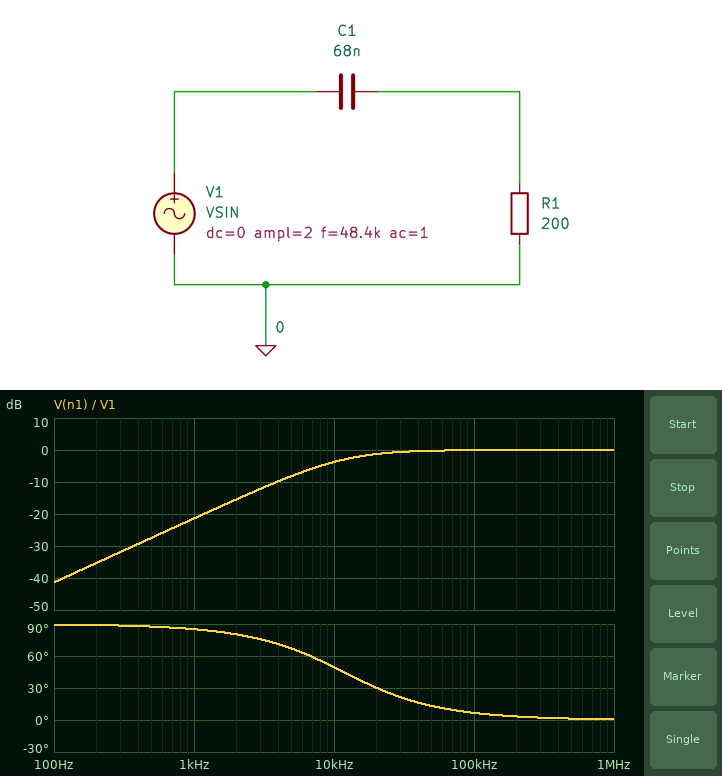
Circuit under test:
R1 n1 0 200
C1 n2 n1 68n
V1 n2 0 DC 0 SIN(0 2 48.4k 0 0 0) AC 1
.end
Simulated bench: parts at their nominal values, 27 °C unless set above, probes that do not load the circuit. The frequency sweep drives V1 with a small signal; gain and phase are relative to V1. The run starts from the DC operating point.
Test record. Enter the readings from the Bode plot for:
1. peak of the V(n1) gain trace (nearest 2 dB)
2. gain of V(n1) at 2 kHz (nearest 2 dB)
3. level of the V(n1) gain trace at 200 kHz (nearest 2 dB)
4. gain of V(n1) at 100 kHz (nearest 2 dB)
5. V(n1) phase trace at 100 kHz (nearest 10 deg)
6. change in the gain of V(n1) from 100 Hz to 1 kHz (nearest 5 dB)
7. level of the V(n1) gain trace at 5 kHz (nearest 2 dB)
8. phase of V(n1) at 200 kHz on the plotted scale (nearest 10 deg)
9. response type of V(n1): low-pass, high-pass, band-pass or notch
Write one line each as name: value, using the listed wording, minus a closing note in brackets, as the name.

peak of the V(n1) gain trace: 0 dB
gain of V(n1) at 2 kHz: -16 dB
level of the V(n1) gain trace at 200 kHz: 0 dB
gain of V(n1) at 100 kHz: 0 dB
V(n1) phase trace at 100 kHz: 10 deg
change in the gain of V(n1) from 100 Hz to 1 kHz: 20 dB
level of the V(n1) gain trace at 5 kHz: -8 dB
phase of V(n1) at 200 kHz on the plotted scale: 0 deg
response type of V(n1): low-pass, high-pass, band-pass or notch: high-pass
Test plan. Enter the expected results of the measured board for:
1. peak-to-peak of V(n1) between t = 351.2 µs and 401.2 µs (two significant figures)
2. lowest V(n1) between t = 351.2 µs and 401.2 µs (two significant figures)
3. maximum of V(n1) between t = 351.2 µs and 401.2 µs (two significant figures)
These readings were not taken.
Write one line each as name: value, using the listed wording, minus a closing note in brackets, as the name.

peak-to-peak of V(n1) between t = 351.2 µs and 401.2 µs: 3.9 V
lowest V(n1) between t = 351.2 µs and 401.2 µs: -1.9 V
maximum of V(n1) between t = 351.2 µs and 401.2 µs: 1.9 V
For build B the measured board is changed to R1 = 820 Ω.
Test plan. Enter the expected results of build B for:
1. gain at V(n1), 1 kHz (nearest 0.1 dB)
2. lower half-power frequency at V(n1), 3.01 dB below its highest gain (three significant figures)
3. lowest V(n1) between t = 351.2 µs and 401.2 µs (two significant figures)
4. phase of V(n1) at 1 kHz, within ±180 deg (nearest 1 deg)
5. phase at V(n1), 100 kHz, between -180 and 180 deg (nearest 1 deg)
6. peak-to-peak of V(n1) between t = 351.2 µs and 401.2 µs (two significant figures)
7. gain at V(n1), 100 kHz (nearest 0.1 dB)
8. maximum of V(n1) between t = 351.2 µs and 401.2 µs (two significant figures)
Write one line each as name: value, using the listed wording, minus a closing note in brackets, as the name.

gain at V(n1), 1 kHz: -9.6 dB
lower half-power frequency at V(n1), 3.01 dB below its highest gain: 2.85 kHz
lowest V(n1) between t = 351.2 µs and 401.2 µs: -2.0 V
phase of V(n1) at 1 kHz, within ±180 deg: 71 deg
phase at V(n1), 100 kHz, between -180 and 180 deg: 2 deg
peak-to-peak of V(n1) between t = 351.2 µs and 401.2 µs: 4.0 V
gain at V(n1), 100 kHz: 0 dB
maximum of V(n1) between t = 351.2 µs and 401.2 µs: 2.0 V
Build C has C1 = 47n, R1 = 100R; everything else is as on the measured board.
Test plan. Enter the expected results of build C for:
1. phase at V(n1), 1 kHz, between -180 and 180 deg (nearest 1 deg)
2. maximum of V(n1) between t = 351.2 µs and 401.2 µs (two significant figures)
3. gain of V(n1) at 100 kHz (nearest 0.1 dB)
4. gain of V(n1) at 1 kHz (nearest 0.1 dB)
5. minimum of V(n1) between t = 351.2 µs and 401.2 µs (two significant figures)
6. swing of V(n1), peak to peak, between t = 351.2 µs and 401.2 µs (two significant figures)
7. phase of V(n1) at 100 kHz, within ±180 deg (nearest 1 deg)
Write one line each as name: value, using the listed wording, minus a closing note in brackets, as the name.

phase at V(n1), 1 kHz, between -180 and 180 deg: 88 deg
maximum of V(n1) between t = 351.2 µs and 401.2 µs: 1.6 V
gain of V(n1) at 100 kHz: -0.5 dB
gain of V(n1) at 1 kHz: -30.6 dB
minimum of V(n1) between t = 351.2 µs and 401.2 µs: -1.6 V
swing of V(n1), peak to peak, between t = 351.2 µs and 401.2 µs: 3.3 V
phase of V(n1) at 100 kHz, within ±180 deg: 19 deg
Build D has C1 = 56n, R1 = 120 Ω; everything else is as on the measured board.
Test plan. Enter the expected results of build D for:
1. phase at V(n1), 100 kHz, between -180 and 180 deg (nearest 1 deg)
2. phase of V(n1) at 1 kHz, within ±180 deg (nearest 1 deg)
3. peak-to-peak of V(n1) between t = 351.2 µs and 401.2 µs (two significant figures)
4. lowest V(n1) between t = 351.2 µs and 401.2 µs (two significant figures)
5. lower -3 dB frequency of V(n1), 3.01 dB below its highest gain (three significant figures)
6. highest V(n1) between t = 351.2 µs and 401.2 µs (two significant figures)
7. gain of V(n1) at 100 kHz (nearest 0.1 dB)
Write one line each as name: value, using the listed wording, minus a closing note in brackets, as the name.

phase at V(n1), 100 kHz, between -180 and 180 deg: 13 deg
phase of V(n1) at 1 kHz, within ±180 deg: 88 deg
peak-to-peak of V(n1) between t = 351.2 µs and 401.2 µs: 3.6 V
lowest V(n1) between t = 351.2 µs and 401.2 µs: -1.8 V
lower -3 dB frequency of V(n1), 3.01 dB below its highest gain: 23.7 kHz
highest V(n1) between t = 351.2 µs and 401.2 µs: 1.8 V
gain of V(n1) at 100 kHz: -0.2 dB
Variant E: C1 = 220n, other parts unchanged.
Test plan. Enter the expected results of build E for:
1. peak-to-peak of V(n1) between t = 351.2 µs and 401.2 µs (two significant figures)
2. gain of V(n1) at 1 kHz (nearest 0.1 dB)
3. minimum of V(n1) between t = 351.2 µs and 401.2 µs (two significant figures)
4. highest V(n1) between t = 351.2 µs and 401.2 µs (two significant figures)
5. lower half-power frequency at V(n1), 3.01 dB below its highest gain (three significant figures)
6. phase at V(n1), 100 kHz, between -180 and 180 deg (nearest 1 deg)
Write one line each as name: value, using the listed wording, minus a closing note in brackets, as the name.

peak-to-peak of V(n1) between t = 351.2 µs and 401.2 µs: 4.0 V
gain of V(n1) at 1 kHz: -11.5 dB
minimum of V(n1) between t = 351.2 µs and 401.2 µs: -2.0 V
highest V(n1) between t = 351.2 µs and 401.2 µs: 2.0 V
lower half-power frequency at V(n1), 3.01 dB below its highest gain: 3.62 kHz
phase at V(n1), 100 kHz, between -180 and 180 deg: 2 deg
